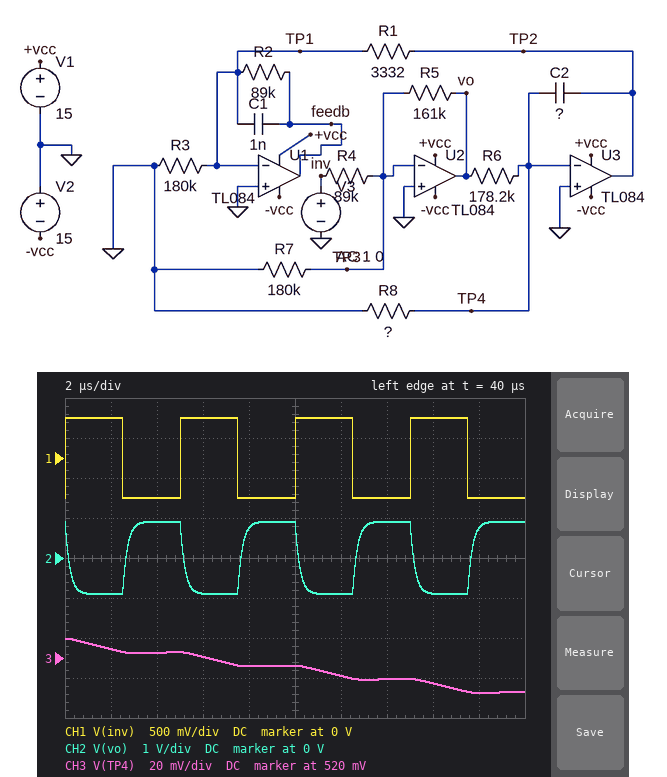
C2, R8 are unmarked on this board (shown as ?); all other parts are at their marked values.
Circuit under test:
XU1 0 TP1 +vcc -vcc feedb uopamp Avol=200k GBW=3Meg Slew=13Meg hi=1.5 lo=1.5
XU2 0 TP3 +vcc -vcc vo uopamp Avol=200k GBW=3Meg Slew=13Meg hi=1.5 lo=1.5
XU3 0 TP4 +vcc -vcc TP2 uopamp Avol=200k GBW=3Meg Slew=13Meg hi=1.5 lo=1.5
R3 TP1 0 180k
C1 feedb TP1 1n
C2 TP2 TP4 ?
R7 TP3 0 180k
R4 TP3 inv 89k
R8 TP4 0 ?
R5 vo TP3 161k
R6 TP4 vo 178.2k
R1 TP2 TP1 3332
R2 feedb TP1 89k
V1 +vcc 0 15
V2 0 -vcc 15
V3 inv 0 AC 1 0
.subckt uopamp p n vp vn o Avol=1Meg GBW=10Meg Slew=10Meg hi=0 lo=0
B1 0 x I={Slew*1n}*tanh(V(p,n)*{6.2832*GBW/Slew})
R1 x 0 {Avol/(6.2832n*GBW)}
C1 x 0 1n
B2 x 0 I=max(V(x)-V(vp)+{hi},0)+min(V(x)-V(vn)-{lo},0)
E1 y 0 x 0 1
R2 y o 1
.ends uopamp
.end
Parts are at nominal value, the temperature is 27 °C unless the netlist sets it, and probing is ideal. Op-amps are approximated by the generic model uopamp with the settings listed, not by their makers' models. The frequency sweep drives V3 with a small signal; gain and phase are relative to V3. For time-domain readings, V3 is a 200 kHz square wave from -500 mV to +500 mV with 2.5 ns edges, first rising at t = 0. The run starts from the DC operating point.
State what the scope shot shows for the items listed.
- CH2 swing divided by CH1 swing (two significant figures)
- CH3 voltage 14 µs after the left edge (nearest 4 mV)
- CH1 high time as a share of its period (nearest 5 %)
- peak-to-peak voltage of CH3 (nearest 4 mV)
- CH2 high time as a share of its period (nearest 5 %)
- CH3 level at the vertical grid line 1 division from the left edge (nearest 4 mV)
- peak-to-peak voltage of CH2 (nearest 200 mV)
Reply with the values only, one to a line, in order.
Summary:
1.8
508 mV
50 %
28 mV
50 %
524 mV
1.8 V
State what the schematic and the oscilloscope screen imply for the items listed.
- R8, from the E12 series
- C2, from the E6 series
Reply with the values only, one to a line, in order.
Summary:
330 kΩ
3.3 nF
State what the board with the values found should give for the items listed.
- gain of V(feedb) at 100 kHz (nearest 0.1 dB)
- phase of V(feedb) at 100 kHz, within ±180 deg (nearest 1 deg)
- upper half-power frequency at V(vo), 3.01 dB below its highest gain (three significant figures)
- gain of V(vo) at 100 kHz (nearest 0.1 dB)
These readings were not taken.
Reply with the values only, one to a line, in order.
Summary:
-52.8 dB
-10 deg
810 kHz
5.1 dB
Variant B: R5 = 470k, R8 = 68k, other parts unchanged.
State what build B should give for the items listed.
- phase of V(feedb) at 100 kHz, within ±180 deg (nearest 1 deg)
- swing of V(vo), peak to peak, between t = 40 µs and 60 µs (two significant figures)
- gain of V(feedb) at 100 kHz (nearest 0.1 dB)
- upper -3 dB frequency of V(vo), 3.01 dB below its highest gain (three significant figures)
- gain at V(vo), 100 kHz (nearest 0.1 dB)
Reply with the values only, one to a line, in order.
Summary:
-19 deg
5.2 V
-43.8 dB
337 kHz
14.1 dB
